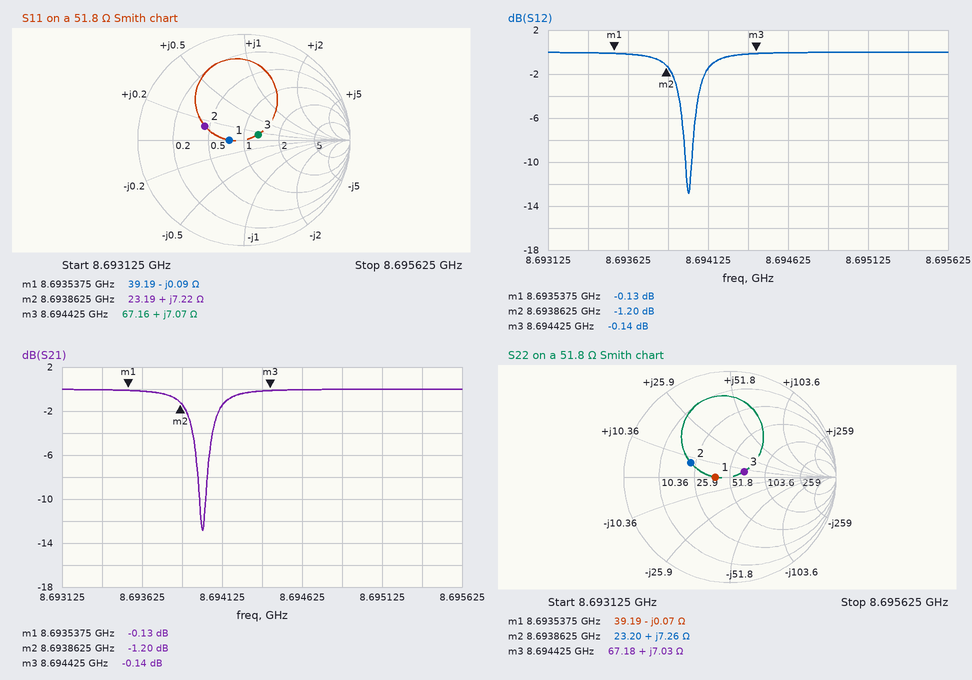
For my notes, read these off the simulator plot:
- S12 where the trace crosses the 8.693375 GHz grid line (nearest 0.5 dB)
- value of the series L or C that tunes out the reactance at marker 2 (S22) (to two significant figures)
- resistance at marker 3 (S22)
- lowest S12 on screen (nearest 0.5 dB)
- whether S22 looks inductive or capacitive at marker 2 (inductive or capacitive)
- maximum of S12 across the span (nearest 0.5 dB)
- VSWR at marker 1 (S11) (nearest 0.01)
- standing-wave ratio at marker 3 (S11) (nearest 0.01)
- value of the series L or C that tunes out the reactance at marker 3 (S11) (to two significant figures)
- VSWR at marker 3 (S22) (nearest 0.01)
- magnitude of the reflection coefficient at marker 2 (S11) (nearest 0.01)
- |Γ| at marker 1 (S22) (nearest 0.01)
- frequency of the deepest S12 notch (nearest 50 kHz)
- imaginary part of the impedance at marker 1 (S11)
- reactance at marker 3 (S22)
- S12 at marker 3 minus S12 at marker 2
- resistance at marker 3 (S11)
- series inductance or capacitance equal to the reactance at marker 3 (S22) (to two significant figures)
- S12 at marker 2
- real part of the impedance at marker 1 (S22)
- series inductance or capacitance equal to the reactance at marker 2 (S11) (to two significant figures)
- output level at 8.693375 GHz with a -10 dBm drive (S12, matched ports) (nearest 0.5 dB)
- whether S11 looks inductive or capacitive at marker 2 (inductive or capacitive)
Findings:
0.0 dB
2.5 pF
67.18 Ω
-13.0 dB
inductive
0.0 dB
1.32
1.33
2.6 pF
1.33
0.39
0.14
8.69400 GHz
-0.09 Ω
+7.03 Ω
1.06 dB
67.16 Ω
130 pH
-1.20 dB
39.19 Ω
130 pH
-10.0 dBm
inductive
